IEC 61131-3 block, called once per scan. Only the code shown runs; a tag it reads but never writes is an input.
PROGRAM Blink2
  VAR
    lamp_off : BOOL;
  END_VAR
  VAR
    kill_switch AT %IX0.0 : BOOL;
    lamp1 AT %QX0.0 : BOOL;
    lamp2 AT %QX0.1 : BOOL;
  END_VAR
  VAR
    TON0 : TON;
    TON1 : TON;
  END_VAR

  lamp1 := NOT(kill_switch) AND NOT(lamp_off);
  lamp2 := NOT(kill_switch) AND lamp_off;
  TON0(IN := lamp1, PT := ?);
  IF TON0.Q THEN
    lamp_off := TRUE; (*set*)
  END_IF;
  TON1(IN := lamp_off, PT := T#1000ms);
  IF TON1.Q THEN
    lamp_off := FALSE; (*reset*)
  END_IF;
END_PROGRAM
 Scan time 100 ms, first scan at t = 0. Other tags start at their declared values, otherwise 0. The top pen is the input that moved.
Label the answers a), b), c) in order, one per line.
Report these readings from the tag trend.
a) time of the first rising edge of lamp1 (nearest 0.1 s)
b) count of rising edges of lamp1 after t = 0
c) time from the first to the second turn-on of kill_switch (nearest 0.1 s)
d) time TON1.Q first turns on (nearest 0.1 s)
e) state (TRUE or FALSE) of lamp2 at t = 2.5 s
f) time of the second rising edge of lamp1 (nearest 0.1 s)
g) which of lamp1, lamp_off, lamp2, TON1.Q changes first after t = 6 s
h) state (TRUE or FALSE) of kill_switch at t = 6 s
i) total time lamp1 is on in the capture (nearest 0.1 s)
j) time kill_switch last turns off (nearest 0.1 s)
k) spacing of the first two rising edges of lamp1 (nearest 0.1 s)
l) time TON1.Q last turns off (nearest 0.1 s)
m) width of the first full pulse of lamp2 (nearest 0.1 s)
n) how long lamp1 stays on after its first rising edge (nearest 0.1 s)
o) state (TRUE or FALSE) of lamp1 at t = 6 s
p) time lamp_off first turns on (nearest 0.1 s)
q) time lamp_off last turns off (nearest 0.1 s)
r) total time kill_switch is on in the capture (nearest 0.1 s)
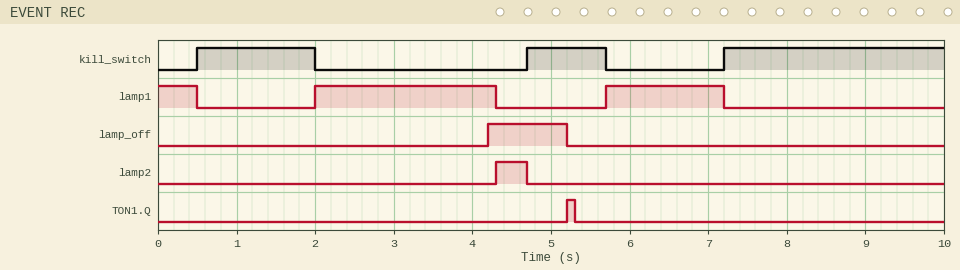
a) 2.0 s
b) 2
c) 4.2 s
d) 5.2 s
e) FALSE
f) 5.7 s
g) lamp1
h) FALSE
i) 4.3 s
j) 5.7 s
k) 3.7 s
l) 5.3 s
m) 0.4 s
n) 2.3 s
o) TRUE
p) 4.2 s
q) 5.2 s
r) 5.3 s
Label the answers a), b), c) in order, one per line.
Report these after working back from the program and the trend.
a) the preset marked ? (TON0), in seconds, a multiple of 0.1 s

a) 2.2 s
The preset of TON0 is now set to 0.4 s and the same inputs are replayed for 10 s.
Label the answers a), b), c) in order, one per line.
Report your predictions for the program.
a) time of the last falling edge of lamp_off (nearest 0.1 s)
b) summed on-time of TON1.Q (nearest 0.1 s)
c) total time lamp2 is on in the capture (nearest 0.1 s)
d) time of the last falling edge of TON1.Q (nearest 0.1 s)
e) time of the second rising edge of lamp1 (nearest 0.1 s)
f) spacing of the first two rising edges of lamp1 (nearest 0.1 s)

a) 7.1 s
b) 0.4 s
c) 2.7 s
d) 7.2 s
e) 3.5 s
f) 1.5 s
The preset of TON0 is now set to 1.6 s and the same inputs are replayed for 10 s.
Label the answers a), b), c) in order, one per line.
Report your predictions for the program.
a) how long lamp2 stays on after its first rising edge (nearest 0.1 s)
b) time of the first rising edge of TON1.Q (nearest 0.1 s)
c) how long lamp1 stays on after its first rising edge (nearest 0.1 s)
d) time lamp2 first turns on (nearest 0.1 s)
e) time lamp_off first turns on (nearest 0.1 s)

a) 1.0 s
b) 4.6 s
c) 1.7 s
d) 3.7 s
e) 3.6 s
